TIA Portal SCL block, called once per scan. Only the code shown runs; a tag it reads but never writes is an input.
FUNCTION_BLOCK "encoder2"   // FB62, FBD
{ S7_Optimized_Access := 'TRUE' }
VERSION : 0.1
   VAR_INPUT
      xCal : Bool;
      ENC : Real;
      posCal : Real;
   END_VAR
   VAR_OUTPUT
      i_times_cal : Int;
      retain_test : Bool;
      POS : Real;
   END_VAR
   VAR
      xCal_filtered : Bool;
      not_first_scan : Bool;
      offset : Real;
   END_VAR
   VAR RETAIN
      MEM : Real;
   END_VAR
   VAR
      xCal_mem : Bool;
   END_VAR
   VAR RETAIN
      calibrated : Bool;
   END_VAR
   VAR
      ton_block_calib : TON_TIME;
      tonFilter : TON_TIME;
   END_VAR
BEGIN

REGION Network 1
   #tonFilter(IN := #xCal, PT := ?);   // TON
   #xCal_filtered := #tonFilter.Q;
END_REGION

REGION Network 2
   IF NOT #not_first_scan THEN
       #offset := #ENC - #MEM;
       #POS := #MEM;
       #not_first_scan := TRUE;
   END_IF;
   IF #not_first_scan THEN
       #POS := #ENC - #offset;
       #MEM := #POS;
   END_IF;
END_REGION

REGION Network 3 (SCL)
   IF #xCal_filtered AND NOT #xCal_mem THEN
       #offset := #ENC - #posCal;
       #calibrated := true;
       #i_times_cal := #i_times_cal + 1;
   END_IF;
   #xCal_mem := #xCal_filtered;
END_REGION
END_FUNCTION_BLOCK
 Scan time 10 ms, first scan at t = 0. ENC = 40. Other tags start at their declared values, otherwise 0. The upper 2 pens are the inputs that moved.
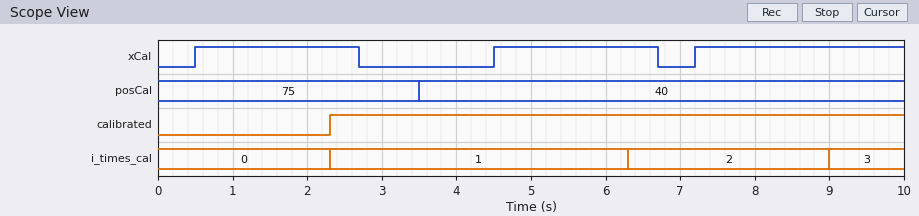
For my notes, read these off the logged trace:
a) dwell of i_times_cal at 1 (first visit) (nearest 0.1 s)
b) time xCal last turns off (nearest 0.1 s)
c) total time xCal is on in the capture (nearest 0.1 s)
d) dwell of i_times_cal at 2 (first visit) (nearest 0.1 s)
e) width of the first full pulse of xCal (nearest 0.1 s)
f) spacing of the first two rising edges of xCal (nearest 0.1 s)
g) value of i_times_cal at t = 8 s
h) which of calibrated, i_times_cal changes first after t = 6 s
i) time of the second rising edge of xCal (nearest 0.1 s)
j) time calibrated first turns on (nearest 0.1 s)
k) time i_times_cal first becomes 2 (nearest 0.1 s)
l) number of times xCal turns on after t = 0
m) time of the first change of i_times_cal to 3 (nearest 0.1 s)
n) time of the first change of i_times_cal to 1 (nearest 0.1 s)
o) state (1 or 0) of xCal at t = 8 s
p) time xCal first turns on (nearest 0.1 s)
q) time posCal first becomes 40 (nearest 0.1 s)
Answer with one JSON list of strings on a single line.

["4.0 s", "6.7 s", "7.2 s", "2.7 s", "2.2 s", "4.0 s", "2", "i_times_cal", "4.5 s", "2.3 s", "6.3 s", "3", "9.0 s", "2.3 s", "1", "0.5 s", "3.5 s"]
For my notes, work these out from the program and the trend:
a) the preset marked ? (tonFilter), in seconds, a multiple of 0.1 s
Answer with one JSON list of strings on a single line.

["1.8 s"]
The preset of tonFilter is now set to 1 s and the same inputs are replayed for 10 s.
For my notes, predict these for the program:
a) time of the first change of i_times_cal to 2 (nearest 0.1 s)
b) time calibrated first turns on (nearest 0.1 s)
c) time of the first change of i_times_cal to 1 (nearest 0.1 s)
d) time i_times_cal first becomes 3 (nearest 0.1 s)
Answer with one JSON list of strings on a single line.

["5.5 s", "1.5 s", "1.5 s", "8.2 s"]
